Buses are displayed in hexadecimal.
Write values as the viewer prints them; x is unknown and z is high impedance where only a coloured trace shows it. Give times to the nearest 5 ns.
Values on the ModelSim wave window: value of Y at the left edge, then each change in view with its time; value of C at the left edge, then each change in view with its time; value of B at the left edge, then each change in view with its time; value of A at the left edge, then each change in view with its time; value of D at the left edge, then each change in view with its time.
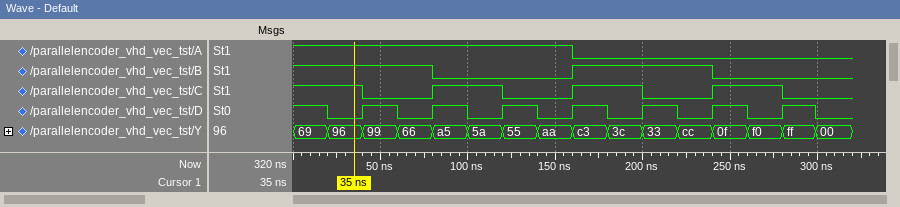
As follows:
69, 96 at 20 ns, 99 at 40 ns, 66 at 60 ns, a5 at 80 ns, 5a at 100 ns, 55 at 120 ns, aa at 140 ns, c3 at 160 ns, 3c at 180 ns, 33 at 200 ns, cc at 220 ns, 0f at 240 ns, f0 at 260 ns, ff at 280 ns, 00 at 300 ns
1, 0 at 40 ns, 1 at 80 ns, 0 at 120 ns, 1 at 160 ns, 0 at 200 ns, 1 at 240 ns, 0 at 280 ns
1, 0 at 80 ns, 1 at 160 ns, 0 at 240 ns
1, 0 at 160 ns
1, 0 at 20 ns, 1 at 40 ns, 0 at 60 ns, 1 at 80 ns, 0 at 100 ns, 1 at 120 ns, 0 at 140 ns, 1 at 160 ns, 0 at 180 ns, 1 at 200 ns, 0 at 220 ns, 1 at 240 ns, 0 at 260 ns, 1 at 280 ns, 0 at 300 ns
